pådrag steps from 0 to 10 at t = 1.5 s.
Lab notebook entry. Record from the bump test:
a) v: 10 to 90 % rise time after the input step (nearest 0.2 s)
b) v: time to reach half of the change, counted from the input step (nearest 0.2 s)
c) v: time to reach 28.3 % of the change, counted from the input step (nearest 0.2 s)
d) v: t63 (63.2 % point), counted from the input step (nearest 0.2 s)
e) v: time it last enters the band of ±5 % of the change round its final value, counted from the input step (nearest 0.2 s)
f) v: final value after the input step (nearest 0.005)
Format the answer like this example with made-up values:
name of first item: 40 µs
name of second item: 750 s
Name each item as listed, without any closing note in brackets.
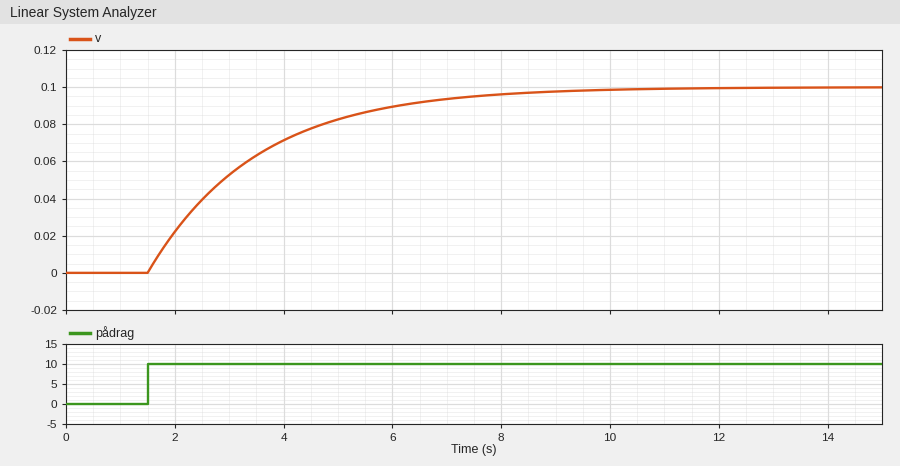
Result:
v: 10 to 90 % rise time after the input step: 4.4 s
v: time to reach half of the change, counted from the input step: 1.4 s
v: time to reach 28.3 % of the change, counted from the input step: 0.6 s
v: t63 (63.2 % point), counted from the input step: 2.0 s
v: time it last enters the band of ±5 % of the change round its final value, counted from the input step: 6.0 s
v: final value after the input step: 0.100
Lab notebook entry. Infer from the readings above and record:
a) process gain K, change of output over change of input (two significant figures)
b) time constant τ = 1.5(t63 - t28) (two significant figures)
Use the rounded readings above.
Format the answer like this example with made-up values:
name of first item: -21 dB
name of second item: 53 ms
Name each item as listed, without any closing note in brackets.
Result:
process gain K, change of output over change of input: 0.010
time constant τ = 1.5(t63 - t28): 2.1 s
